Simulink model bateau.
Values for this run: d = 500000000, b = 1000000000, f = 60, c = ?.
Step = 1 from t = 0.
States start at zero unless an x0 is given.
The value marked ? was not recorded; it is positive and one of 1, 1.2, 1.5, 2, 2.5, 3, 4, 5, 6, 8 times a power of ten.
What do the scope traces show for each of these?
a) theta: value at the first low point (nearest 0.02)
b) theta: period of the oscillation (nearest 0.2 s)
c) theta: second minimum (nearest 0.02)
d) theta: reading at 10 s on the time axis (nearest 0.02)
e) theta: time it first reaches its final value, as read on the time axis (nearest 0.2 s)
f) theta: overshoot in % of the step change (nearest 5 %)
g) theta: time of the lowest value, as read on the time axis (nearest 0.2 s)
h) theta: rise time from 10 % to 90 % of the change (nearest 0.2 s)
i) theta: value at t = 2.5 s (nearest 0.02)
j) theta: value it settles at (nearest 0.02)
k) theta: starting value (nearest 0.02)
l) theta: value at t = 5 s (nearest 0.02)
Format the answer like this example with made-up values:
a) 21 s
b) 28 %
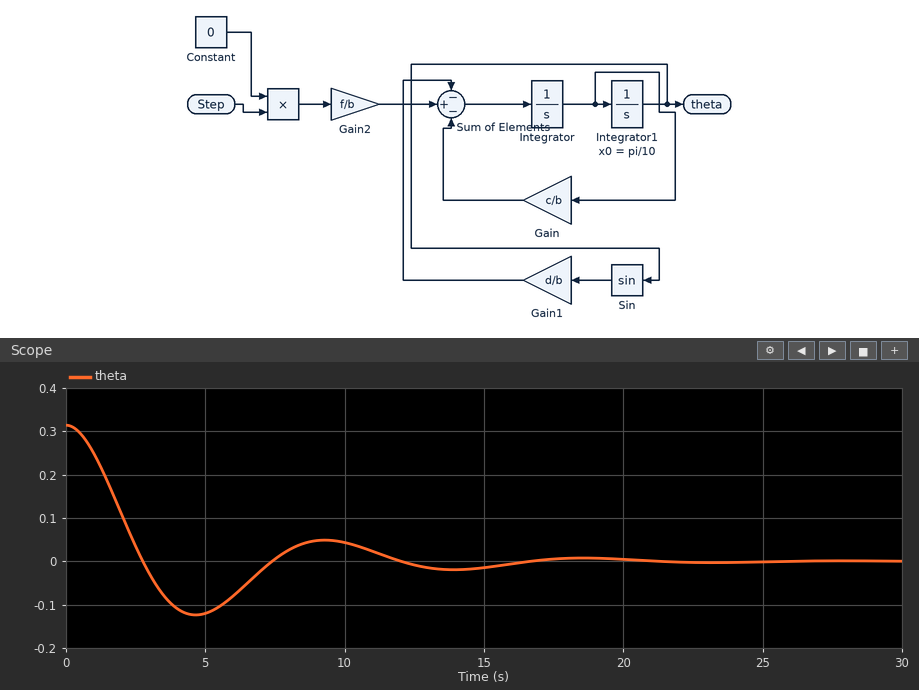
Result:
a) -0.12
b) 9.2 s
c) -0.02
d) 0.04
e) 2.8 s
f) 40 %
g) 4.6 s
h) 1.8 s
i) 0.04
j) 0.00
k) 0.32
l) -0.12
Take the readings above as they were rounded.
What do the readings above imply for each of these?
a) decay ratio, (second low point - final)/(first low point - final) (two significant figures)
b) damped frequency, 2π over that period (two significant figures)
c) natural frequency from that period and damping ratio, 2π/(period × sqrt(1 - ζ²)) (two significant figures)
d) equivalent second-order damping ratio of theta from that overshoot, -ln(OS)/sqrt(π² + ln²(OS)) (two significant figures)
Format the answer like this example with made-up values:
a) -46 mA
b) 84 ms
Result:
a) 0.17
b) 0.68 rad/s
c) 0.71 rad/s
d) 0.28
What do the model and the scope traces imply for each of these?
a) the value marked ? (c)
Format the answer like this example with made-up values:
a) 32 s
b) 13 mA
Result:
a) 4e+08
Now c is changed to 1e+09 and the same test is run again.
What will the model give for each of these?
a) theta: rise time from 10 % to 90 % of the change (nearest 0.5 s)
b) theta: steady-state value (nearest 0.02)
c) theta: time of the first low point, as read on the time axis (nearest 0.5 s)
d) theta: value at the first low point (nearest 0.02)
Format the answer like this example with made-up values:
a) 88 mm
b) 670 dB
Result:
a) 3.0 s
b) 0.00
c) 6.5 s
d) -0.02
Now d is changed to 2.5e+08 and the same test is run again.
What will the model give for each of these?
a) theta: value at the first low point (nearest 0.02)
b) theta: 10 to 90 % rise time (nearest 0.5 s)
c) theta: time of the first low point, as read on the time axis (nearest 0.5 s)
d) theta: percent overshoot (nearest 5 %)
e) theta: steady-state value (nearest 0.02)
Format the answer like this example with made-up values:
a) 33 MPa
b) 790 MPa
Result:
a) -0.08
b) 3.0 s
c) 7.0 s
d) 25 %
e) 0.00
